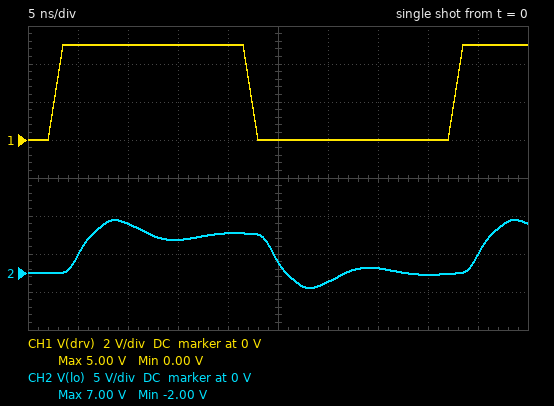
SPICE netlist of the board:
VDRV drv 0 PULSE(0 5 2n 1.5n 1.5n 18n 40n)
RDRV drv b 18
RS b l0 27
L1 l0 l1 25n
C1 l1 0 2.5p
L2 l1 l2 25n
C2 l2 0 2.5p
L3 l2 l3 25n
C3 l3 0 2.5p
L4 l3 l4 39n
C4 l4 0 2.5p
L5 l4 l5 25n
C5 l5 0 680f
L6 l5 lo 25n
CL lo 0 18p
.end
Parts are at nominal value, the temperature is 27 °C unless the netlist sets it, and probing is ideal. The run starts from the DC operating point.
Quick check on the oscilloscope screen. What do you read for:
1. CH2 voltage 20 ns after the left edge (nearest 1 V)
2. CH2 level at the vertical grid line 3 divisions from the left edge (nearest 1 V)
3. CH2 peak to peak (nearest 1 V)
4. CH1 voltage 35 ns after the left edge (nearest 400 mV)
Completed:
5 V
4 V
9 V
0 V
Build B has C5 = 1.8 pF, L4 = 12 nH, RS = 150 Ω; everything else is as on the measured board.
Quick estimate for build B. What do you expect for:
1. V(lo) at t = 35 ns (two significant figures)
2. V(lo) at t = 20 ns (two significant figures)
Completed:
310 mV
4.9 V
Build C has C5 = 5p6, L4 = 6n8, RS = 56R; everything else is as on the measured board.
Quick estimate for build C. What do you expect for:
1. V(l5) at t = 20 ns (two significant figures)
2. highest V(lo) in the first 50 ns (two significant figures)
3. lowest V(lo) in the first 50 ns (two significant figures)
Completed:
5.0 V
5.3 V
-280 mV
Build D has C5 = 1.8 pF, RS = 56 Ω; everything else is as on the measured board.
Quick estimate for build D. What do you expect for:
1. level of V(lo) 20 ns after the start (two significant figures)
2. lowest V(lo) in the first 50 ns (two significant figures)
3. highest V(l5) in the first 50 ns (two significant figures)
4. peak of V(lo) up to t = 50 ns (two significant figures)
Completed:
5.0 V
-670 mV
5.6 V
5.7 V
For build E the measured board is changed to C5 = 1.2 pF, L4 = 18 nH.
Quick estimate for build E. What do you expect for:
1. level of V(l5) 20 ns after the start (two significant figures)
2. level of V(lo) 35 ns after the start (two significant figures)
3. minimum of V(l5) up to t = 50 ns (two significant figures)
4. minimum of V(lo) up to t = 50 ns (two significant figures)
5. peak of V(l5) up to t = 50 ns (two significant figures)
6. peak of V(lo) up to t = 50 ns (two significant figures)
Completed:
5.1 V
400 mV
-1.4 V
-1.8 V
6.4 V
6.8 V
